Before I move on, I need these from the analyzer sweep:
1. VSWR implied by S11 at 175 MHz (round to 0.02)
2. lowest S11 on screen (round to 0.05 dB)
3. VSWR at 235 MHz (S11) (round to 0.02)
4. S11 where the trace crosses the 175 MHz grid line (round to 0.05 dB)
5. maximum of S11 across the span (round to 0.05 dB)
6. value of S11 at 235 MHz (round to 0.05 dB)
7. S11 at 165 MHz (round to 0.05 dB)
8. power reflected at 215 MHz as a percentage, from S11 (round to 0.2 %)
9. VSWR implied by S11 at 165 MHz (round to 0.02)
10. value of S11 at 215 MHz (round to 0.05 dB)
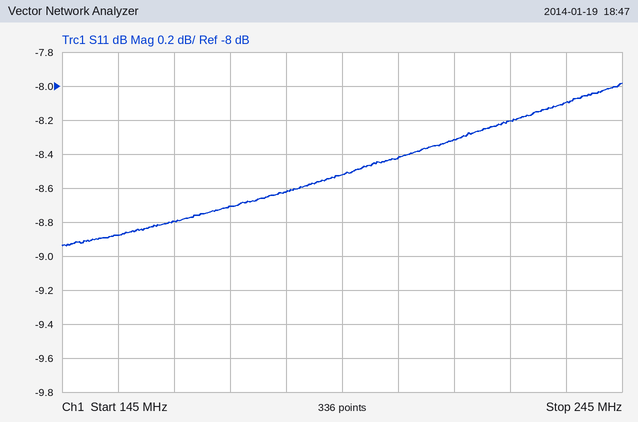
2.16
-8.95 dB
2.30
-8.70 dB
-8.00 dB
-8.10 dB
-8.80 dB
14.8 %
2.14
-8.30 dB
